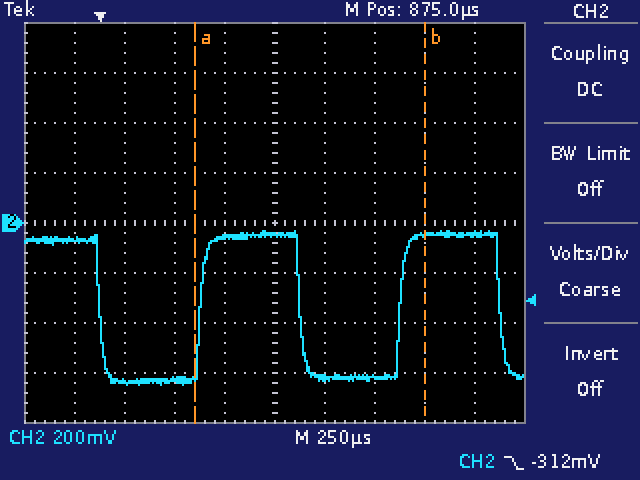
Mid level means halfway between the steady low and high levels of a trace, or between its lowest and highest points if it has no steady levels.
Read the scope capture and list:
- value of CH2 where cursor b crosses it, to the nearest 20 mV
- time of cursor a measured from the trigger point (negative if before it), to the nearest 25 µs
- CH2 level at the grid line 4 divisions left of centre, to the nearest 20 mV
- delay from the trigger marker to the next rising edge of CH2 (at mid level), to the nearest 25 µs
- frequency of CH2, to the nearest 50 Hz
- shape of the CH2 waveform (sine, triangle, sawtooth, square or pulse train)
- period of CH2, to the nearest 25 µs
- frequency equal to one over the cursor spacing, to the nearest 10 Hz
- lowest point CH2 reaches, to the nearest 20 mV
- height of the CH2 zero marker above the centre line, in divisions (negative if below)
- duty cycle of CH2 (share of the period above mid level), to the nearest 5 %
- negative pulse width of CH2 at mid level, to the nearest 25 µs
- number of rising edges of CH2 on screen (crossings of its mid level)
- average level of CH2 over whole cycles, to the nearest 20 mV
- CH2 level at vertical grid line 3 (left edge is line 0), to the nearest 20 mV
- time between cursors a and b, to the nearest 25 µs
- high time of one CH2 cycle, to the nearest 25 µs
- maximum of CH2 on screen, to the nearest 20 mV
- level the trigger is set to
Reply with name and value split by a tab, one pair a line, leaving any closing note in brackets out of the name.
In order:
value of CH2 where cursor b crosses it, to the nearest 20 mV	-40 mV
time of cursor a measured from the trigger point (negative if before it), to the nearest 25 µs	+475 µs
CH2 level at the grid line 4 divisions left of centre, to the nearest 20 mV	-60 mV
delay from the trigger marker to the next rising edge of CH2 (at mid level), to the nearest 25 µs	500 µs
frequency of CH2, to the nearest 50 Hz	1.00 kHz
shape of the CH2 waveform	square
period of CH2, to the nearest 25 µs	1.000 ms
frequency equal to one over the cursor spacing, to the nearest 10 Hz	870 Hz
lowest point CH2 reaches, to the nearest 20 mV	-640 mV
height of the CH2 zero marker above the centre line, in divisions	0.0 div
duty cycle of CH2 (share of the period above mid level), to the nearest 5 %	50 %
negative pulse width of CH2 at mid level, to the nearest 25 µs	500 µs
number of rising edges of CH2 on screen	2
average level of CH2 over whole cycles, to the nearest 20 mV	-340 mV
CH2 level at vertical grid line 3 (left edge is line 0), to the nearest 20 mV	-620 mV
time between cursors a and b, to the nearest 25 µs	1.150 ms
high time of one CH2 cycle, to the nearest 25 µs	500 µs
maximum of CH2 on screen, to the nearest 20 mV	-40 mV
level the trigger is set to	-312 mV
